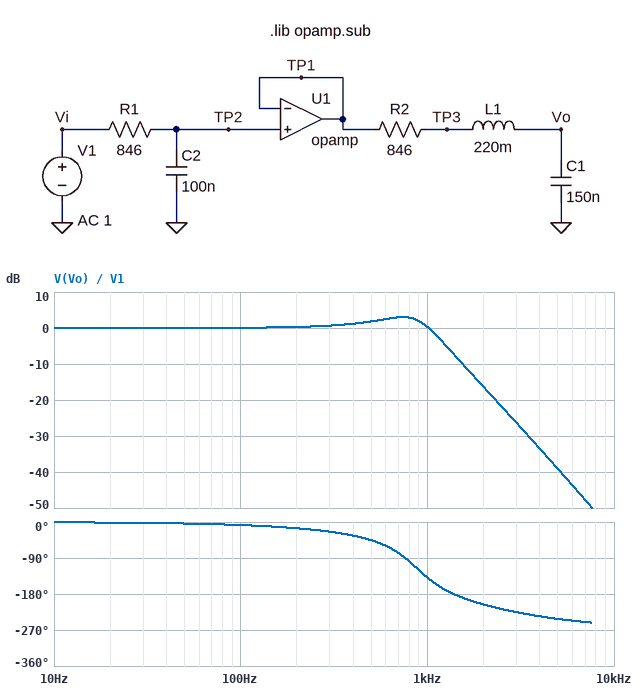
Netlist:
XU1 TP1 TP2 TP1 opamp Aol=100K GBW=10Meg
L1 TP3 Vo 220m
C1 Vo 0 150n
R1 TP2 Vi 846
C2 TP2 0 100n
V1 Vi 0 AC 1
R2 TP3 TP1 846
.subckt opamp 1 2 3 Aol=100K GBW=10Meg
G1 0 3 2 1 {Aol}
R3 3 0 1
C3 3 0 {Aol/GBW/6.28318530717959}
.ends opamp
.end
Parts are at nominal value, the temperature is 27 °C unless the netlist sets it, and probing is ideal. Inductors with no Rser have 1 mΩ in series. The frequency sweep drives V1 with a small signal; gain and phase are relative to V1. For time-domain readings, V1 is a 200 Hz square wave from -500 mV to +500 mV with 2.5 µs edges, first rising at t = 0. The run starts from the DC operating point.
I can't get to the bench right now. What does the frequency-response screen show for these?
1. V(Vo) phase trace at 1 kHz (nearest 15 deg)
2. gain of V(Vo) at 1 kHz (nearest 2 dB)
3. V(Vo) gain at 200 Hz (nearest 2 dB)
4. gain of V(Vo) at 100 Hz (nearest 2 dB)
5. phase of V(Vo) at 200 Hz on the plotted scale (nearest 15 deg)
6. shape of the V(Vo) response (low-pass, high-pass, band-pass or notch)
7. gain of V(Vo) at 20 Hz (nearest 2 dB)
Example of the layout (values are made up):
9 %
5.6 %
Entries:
-135 deg
0 dB
0 dB
0 dB
-15 deg
low-pass
0 dB
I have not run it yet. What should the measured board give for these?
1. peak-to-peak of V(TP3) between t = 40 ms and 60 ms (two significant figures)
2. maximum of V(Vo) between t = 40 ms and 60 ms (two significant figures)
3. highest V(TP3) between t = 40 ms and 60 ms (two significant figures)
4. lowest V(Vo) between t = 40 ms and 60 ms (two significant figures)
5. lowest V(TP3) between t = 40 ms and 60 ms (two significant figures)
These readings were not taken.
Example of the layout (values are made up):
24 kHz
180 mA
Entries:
1.2 V
770 mV
620 mV
-770 mV
-620 mV
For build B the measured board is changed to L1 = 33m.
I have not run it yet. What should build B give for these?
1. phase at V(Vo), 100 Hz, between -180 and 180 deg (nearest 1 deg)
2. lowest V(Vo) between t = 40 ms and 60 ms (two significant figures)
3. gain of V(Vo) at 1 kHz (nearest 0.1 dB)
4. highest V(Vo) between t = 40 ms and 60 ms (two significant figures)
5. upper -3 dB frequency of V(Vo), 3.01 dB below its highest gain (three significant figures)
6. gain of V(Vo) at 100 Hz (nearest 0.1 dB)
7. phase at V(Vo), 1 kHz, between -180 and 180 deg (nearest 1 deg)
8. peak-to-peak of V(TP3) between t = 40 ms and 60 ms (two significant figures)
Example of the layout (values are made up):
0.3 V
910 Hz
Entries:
-8 deg
-500 mV
-2.2 dB
500 mV
1.19 kHz
0 dB
-73 deg
1.0 V
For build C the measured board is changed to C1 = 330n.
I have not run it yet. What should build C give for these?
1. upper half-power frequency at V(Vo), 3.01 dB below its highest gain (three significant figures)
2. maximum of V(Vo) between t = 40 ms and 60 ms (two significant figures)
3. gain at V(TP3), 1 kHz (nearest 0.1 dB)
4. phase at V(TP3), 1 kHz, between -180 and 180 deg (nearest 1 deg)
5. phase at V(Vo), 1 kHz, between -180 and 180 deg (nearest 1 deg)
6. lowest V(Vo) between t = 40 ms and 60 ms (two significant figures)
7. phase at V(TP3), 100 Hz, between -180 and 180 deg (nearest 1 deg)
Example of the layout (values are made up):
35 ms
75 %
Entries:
669 Hz
640 mV
-3.8 dB
15 deg
-165 deg
-640 mV
-13 deg
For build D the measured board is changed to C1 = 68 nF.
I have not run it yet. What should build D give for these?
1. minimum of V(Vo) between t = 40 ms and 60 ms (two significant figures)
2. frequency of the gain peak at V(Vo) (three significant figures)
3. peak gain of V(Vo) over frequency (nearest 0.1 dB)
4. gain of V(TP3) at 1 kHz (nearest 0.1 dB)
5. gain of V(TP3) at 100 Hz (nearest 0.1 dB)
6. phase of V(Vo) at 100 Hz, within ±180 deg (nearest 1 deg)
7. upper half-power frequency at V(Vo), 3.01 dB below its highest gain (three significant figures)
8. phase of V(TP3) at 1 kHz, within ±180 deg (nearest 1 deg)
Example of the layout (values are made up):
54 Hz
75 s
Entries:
-870 mV
1.20 kHz
5.3 dB
-3.6 dB
0 dB
-5 deg
1.48 kHz
-69 deg
